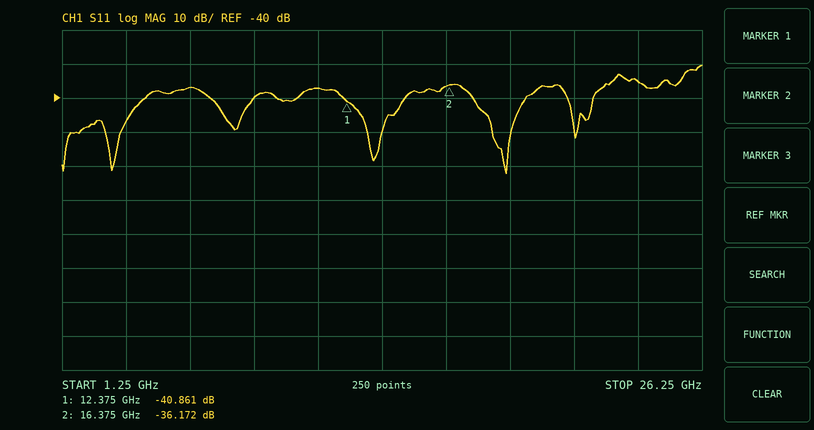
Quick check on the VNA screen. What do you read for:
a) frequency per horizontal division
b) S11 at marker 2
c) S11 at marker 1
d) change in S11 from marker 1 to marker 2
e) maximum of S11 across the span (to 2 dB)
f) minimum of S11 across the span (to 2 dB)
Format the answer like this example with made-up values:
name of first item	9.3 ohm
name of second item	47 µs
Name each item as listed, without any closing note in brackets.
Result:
frequency per horizontal division	2.5 GHz
S11 at marker 2	-36.172 dB
S11 at marker 1	-40.861 dB
change in S11 from marker 1 to marker 2	4.689 dB
maximum of S11 across the span	-30 dB
minimum of S11 across the span	-62 dB
